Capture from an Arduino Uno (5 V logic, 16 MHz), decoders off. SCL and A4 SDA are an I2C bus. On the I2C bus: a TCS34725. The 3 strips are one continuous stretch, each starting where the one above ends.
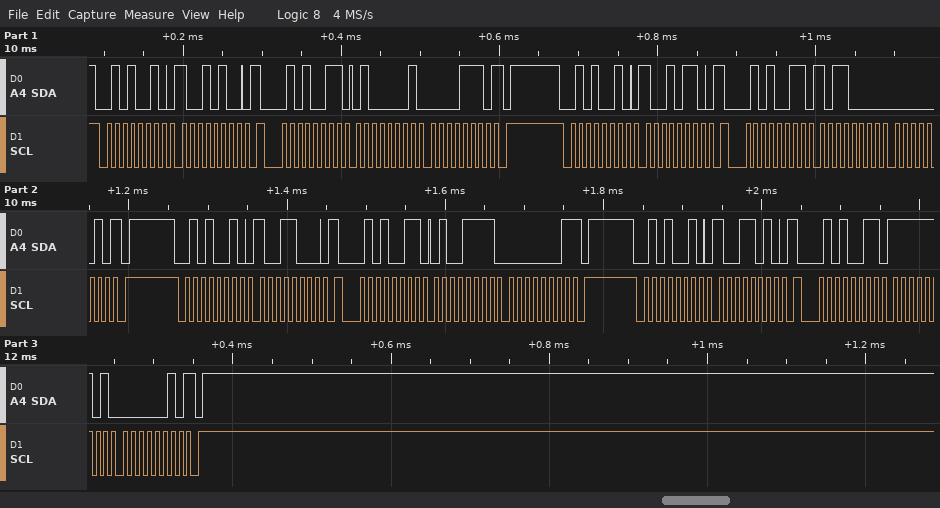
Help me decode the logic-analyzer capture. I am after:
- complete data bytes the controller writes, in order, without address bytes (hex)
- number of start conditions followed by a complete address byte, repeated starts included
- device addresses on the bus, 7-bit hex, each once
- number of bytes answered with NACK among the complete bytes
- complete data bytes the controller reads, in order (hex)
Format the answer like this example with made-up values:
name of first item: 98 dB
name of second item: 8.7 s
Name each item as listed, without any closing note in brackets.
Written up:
complete data bytes the controller writes, in order, without address bytes: 94 96 98 9A
number of start conditions followed by a complete address byte, repeated starts included: 8
device addresses on the bus, 7-bit hex, each once: 0x29
number of bytes answered with NACK among the complete bytes: 4
complete data bytes the controller reads, in order: 41 0E B0 02 4F 01 FD 02
